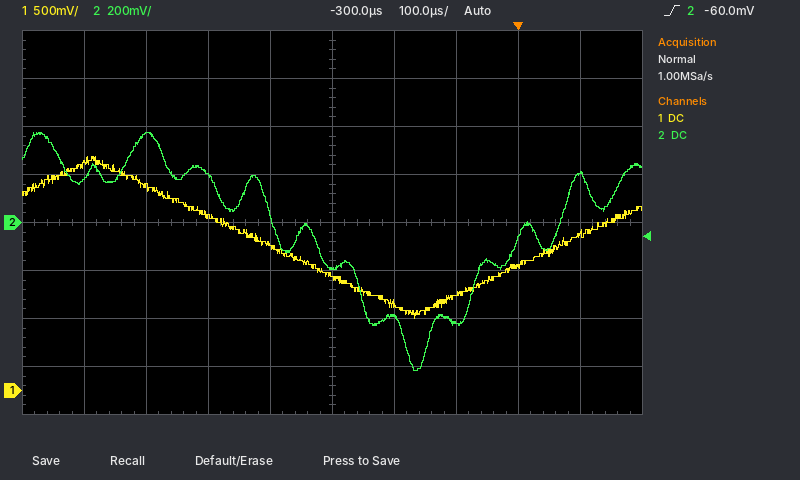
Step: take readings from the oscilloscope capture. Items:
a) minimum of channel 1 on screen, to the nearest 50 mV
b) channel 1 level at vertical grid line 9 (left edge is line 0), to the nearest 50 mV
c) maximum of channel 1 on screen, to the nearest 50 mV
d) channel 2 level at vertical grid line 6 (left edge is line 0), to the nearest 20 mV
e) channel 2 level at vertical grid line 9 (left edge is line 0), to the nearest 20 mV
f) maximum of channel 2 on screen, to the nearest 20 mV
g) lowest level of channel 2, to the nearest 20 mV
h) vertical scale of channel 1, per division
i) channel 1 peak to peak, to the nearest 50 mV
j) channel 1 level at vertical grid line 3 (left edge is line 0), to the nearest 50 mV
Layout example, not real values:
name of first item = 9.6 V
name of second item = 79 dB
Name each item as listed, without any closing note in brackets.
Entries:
minimum of channel 1 on screen, to the nearest 50 mV = 750 mV
channel 1 level at vertical grid line 9 (left edge is line 0), to the nearest 50 mV = 1.65 V
maximum of channel 1 on screen, to the nearest 50 mV = 2.45 V
channel 2 level at vertical grid line 6 (left edge is line 0), to the nearest 20 mV = -400 mV
channel 2 level at vertical grid line 9 (left edge is line 0), to the nearest 20 mV = 200 mV
maximum of channel 2 on screen, to the nearest 20 mV = 380 mV
lowest level of channel 2, to the nearest 20 mV = -620 mV
vertical scale of channel 1, per division = 500 mV
channel 1 peak to peak, to the nearest 50 mV = 1.70 V
channel 1 level at vertical grid line 3 (left edge is line 0), to the nearest 50 mV = 1.85 V
